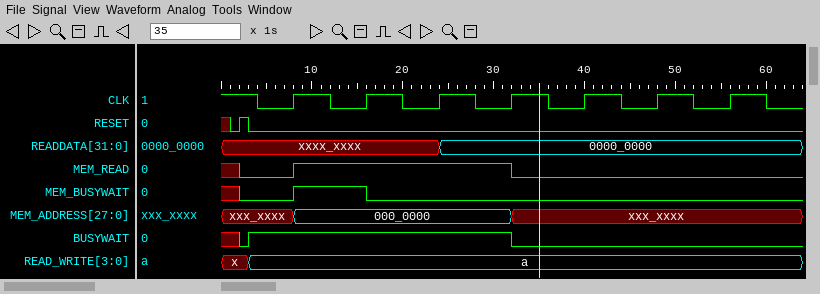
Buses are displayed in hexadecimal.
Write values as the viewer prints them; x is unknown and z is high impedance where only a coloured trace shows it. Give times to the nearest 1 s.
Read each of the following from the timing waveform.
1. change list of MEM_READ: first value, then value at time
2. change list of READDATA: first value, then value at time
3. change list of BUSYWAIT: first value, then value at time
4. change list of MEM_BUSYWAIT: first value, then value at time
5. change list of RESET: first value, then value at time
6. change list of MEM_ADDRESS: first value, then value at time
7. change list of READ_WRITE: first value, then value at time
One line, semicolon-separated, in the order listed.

x, 0 at 2 s, 1 at 8 s, 0 at 32 s; xxxx_xxxx, 0000_0000 at 24 s; x, 0 at 2 s, 1 at 3 s, 0 at 32 s; x, 0 at 2 s, 1 at 8 s, 0 at 16 s; x, 0 at 1 s, 1 at 2 s, 0 at 3 s; xxx_xxxx, 000_0000 at 8 s, xxx_xxxx at 32 s; x, a at 3 s
